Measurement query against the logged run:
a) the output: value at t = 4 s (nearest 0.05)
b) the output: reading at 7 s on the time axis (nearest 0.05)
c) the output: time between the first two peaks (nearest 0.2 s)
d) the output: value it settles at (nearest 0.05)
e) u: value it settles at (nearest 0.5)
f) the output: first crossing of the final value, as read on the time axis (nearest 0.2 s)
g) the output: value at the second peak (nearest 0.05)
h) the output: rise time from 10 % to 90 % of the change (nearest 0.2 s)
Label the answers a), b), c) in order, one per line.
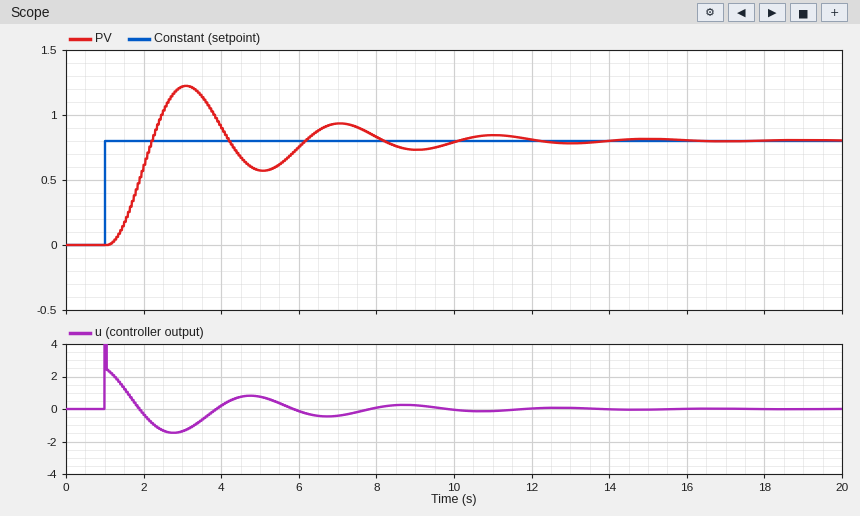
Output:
a) 0.90
b) 0.95
c) 4.0 s
d) 0.80
e) 0.0
f) 2.2 s
g) 0.95
h) 0.8 s
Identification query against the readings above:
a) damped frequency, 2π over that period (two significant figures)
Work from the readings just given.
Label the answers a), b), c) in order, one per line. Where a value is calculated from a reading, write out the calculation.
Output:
a) 2π / 4 = 1.6 rad/s
